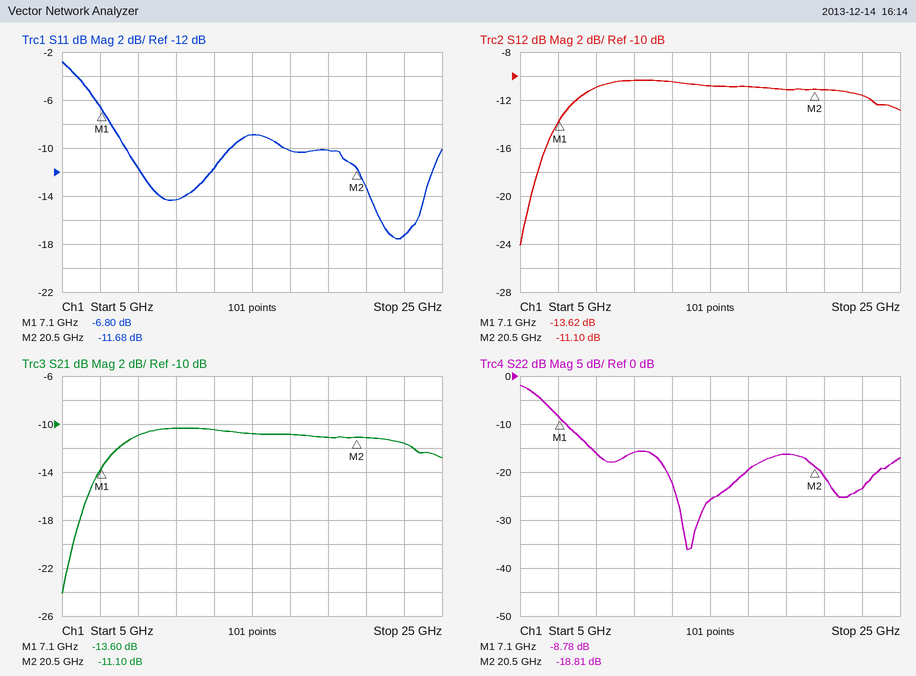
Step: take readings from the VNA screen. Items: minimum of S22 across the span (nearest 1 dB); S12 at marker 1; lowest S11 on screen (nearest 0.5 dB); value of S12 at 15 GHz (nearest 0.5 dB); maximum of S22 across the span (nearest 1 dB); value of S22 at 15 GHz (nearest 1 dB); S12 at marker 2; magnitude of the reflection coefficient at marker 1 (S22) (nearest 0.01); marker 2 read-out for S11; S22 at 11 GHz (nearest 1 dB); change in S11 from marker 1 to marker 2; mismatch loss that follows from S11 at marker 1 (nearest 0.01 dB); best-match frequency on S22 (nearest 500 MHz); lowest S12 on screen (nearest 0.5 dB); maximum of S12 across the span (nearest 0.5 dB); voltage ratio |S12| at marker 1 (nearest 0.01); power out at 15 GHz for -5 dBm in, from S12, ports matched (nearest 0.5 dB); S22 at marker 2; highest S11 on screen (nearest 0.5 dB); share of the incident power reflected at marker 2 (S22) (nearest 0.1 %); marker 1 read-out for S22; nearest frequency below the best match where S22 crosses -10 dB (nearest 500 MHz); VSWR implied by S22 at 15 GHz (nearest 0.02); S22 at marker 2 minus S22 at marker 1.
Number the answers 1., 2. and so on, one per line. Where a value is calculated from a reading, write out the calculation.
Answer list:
1. -36 dB
2. -13.62 dB
3. -17.5 dB
4. -11.0 dB
5. -2 dB
6. -26 dB
7. -11.10 dB
8. 10^(-8.78/20) ≈ 0.36
9. -11.68 dB
10. -16 dB
11. -11.68 − (-6.8) = -4.88 dB
12. −10 log10(1 − 10^(-6.8/10)) ≈ 1.02 dB
13. 14.0 GHz
14. -24.0 dB
15. -10.5 dB
16. 10^(-13.62/20) ≈ 0.21
17. -5 dBm + (-11.0 dB) = -16.0 dBm
18. -18.81 dB
19. -3.0 dB
20. 10^(-18.81/10) ≈ 1.3 %
21. -8.78 dB
22. 7.5 GHz
23. |Γ| = 10^(-26/20) = 0.0501; VSWR = (1 + 0.0501)/(1 − 0.0501) ≈ 1.11, so 1.10 to the nearest 0.02
24. -18.81 − (-8.78) = -10.03 dB
